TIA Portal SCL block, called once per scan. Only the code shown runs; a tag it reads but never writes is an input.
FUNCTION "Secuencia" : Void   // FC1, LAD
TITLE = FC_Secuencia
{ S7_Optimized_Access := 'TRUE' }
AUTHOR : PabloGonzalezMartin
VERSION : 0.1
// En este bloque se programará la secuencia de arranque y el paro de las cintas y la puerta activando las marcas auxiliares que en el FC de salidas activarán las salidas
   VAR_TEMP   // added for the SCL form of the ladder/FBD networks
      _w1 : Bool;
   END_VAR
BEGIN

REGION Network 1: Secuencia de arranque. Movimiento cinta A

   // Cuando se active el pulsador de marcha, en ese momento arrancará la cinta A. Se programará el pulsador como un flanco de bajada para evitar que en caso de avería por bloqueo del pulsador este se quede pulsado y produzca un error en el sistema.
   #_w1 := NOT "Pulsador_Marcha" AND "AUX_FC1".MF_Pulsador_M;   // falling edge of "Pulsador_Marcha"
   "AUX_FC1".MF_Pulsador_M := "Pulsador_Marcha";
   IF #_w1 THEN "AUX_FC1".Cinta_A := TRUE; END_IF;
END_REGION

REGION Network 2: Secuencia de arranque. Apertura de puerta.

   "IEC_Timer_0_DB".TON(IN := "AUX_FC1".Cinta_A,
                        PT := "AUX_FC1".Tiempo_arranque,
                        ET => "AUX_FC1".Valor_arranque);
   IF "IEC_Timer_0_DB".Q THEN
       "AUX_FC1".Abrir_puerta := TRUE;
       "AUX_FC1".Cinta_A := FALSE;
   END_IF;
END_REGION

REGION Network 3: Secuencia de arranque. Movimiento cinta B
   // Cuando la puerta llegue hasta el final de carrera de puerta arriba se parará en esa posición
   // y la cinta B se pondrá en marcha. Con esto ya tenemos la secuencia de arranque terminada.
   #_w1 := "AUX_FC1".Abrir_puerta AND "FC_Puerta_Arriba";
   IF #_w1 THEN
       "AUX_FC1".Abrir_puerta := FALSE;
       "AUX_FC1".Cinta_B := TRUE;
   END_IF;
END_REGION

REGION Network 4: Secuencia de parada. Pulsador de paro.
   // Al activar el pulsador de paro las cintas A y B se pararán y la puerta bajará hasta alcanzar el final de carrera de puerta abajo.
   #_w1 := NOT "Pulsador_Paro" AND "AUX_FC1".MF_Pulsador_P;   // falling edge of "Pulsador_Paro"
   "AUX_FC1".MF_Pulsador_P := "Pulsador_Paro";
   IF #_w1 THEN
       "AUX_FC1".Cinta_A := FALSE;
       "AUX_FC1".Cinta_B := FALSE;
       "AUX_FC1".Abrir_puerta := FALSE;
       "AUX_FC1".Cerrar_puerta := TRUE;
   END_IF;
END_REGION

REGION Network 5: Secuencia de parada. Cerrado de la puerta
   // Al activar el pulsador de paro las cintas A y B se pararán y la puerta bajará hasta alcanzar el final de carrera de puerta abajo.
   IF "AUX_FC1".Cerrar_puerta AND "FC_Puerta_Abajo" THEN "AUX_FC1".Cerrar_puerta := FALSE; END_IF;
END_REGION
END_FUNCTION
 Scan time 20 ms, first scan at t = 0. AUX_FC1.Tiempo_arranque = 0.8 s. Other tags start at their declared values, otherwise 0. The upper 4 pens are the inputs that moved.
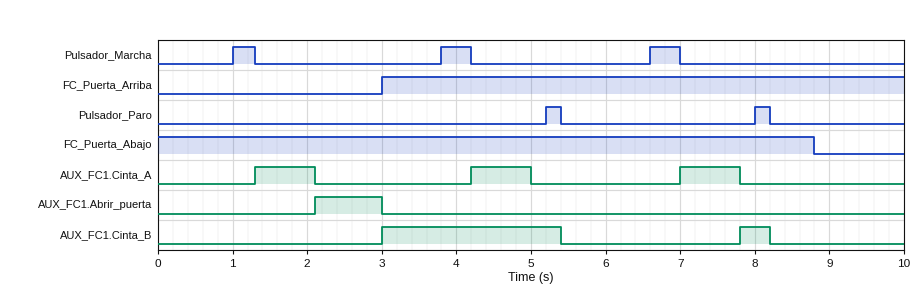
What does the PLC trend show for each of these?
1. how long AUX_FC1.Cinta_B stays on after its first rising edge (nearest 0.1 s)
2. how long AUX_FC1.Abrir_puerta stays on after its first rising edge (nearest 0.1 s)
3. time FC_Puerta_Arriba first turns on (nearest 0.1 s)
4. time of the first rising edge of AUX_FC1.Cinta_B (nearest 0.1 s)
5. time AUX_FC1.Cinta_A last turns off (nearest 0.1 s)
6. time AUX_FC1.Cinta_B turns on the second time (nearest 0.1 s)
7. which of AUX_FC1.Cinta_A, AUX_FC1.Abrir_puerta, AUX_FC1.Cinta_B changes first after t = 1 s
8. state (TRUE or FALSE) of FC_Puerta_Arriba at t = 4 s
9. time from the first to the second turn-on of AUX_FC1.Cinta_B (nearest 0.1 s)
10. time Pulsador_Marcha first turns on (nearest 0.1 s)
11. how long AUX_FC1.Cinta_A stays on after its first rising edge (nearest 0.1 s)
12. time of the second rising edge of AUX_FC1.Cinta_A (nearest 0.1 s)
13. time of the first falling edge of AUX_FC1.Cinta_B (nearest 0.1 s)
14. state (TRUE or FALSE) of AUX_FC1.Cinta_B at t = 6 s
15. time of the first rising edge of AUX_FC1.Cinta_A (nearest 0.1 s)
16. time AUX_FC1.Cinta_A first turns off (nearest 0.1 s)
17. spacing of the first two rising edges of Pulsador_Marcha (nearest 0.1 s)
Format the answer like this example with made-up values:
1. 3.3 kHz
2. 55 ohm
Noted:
1. 2.4 s
2. 0.9 s
3. 3.0 s
4. 3.0 s
5. 7.8 s
6. 7.8 s
7. AUX_FC1.Cinta_A
8. TRUE
9. 4.8 s
10. 1.0 s
11. 0.8 s
12. 4.2 s
13. 5.4 s
14. FALSE
15. 1.3 s
16. 2.1 s
17. 2.8 s
